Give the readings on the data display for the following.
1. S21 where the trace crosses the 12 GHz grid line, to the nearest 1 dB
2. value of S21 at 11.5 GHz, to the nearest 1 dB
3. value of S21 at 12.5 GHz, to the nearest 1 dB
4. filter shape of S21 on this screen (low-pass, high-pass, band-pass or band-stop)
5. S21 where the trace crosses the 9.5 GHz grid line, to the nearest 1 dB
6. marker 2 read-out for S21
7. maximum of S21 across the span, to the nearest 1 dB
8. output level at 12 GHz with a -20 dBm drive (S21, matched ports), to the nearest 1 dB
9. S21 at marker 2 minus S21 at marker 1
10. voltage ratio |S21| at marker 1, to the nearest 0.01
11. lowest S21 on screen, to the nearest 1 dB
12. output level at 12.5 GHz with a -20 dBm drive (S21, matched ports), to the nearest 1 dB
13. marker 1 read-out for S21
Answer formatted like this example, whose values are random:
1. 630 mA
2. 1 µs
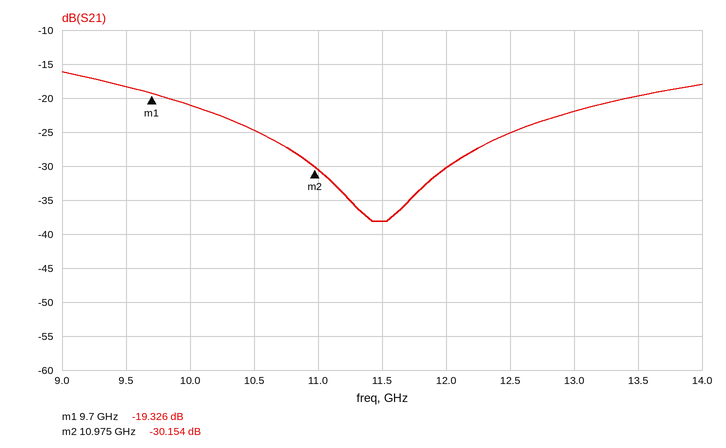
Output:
1. -30 dB
2. -38 dB
3. -25 dB
4. band-stop
5. -18 dB
6. -30.154 dB
7. -16 dB
8. -50 dBm
9. -10.828 dB
10. 0.11
11. -38 dB
12. -45 dBm
13. -19.326 dB
